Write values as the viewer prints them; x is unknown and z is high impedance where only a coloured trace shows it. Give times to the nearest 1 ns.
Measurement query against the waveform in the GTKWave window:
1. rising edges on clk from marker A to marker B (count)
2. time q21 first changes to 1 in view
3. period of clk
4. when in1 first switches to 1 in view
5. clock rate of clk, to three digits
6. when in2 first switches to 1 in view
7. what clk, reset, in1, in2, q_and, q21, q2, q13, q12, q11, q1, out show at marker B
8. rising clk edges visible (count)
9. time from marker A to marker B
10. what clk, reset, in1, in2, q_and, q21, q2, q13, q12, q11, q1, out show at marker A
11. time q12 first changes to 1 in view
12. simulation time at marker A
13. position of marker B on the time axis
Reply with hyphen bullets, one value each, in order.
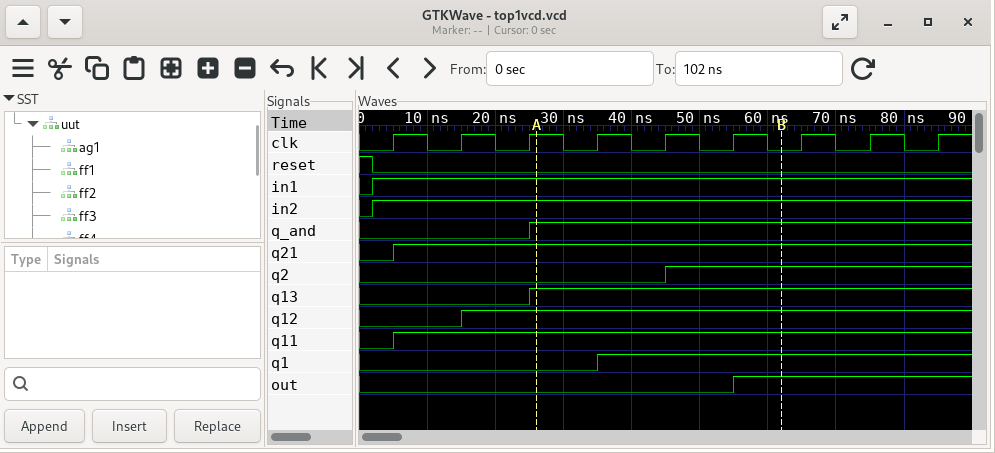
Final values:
- 3
- 5 ns
- 10 ns
- 2 ns
- 100 MHz
- 2 ns
- clk=0, reset=0, in1=1, in2=1, q_and=1, q21=1, q2=1, q13=1, q12=1, q11=1, q1=1, out=1
- 9
- 36 ns
- clk=1, reset=0, in1=1, in2=1, q_and=1, q21=1, q2=0, q13=1, q12=1, q11=1, q1=0, out=0
- 15 ns
- 26 ns
- 62 ns
